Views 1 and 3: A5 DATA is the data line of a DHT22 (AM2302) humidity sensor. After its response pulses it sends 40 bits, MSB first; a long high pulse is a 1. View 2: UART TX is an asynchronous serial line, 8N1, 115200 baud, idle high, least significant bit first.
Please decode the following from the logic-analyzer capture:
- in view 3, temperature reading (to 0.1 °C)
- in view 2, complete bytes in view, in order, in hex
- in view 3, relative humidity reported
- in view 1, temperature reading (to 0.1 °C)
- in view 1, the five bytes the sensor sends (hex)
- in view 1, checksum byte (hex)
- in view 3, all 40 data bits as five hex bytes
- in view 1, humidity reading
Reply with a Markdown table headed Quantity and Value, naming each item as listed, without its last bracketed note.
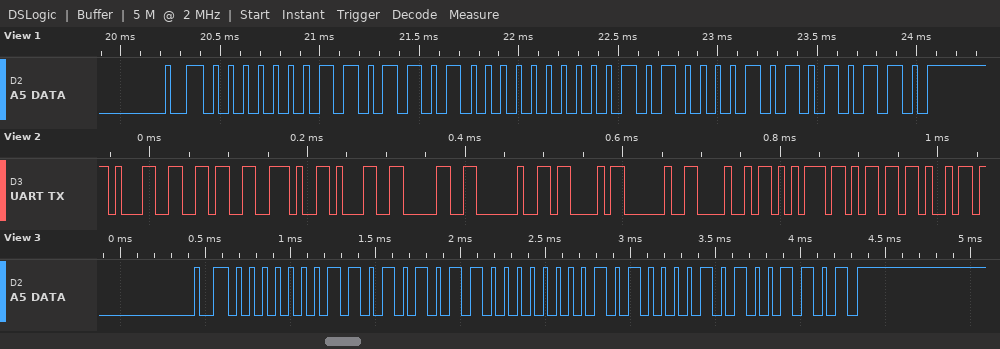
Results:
| Quantity | Value |
|---|---|
| in view 3, temperature reading | 16.1 °C |
| in view 2, complete bytes in view, in order, in hex | 31 36 2E 31 30 20 43 20 48 75 6D 69 |
| in view 3, relative humidity reported | 42.7 % |
| in view 1, temperature reading | 16.1 °C |
| in view 1, the five bytes the sensor sends | 01 B4 00 A1 56 |
| in view 1, checksum byte | 0x56 |
| in view 3, all 40 data bits as five hex bytes | 01 AB 00 A1 4D |
| in view 1, humidity reading | 43.6 % |
